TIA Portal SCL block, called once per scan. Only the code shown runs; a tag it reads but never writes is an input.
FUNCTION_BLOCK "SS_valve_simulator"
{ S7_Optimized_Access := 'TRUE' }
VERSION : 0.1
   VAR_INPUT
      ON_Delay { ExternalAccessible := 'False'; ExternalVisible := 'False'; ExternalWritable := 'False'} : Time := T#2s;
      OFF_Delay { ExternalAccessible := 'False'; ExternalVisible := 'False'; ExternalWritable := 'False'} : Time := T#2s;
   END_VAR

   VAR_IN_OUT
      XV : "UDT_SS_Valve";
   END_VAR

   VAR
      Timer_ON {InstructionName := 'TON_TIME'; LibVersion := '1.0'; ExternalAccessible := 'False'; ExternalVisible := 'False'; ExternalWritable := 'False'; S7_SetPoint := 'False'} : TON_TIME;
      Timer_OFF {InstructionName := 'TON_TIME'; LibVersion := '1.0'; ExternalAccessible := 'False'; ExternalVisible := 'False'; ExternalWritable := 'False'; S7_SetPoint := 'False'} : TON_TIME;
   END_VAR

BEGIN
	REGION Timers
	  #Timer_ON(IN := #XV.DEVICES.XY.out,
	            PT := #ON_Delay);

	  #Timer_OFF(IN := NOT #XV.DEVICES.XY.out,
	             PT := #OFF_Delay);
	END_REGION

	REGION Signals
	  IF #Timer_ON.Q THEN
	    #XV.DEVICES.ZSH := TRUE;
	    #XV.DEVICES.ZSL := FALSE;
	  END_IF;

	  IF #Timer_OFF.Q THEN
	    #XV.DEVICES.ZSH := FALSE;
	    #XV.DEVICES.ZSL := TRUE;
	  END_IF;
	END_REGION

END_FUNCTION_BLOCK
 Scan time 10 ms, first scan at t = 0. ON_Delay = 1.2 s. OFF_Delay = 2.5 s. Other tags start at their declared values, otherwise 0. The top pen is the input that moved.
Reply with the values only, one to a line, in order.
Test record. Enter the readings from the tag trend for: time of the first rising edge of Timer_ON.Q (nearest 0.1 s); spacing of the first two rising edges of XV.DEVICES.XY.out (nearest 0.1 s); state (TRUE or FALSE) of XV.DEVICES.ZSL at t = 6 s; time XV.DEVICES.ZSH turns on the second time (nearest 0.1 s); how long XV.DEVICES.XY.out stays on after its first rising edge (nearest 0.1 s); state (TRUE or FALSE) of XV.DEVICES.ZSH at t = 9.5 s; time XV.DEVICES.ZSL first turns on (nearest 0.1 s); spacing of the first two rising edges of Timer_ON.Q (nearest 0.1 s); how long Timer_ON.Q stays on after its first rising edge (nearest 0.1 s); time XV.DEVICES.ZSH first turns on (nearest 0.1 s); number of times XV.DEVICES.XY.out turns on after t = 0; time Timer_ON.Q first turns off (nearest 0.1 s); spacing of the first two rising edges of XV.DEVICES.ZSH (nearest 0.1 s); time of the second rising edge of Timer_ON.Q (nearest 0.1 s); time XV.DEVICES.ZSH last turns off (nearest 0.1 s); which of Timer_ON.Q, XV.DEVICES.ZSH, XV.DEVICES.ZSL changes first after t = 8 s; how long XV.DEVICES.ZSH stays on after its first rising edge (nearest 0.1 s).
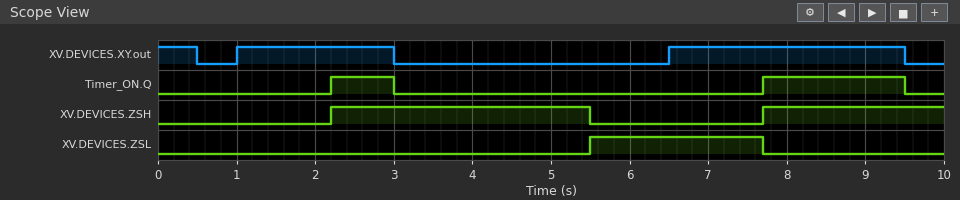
2.2 s
5.5 s
TRUE
7.7 s
2.0 s
TRUE
5.5 s
5.5 s
0.8 s
2.2 s
2
3.0 s
5.5 s
7.7 s
5.5 s
Timer_ON.Q
3.3 s
